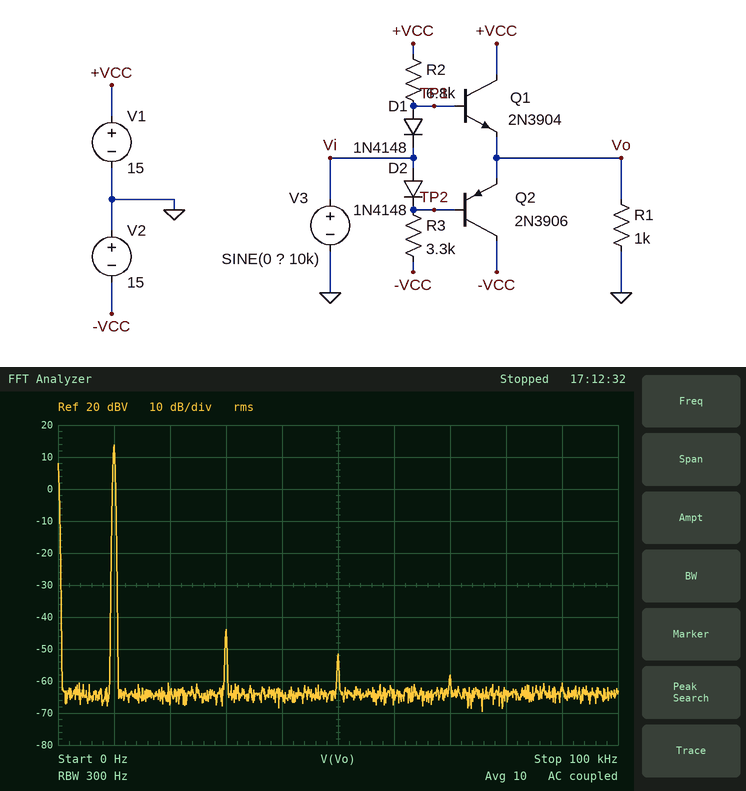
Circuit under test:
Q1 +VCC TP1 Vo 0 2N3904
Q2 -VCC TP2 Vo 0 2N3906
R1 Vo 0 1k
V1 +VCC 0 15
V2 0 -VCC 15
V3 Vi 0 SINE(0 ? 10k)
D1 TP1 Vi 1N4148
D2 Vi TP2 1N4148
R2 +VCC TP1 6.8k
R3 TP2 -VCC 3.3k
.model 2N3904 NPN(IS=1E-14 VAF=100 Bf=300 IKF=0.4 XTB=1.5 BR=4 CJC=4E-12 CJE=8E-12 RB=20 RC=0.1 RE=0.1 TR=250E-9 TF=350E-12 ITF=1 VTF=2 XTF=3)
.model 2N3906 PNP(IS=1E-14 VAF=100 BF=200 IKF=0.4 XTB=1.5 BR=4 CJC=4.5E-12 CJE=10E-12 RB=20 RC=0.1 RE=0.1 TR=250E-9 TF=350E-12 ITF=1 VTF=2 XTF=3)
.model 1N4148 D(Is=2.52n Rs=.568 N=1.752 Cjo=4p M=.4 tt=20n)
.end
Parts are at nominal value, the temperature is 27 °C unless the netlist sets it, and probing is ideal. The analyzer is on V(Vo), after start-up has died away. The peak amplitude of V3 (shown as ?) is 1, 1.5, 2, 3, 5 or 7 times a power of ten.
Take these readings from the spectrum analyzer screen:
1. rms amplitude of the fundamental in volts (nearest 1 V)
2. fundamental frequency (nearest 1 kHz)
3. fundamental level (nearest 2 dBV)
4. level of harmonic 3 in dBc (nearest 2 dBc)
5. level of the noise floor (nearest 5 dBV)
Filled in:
5 V
10 kHz
14 dBV
-58 dBc
-65 dBV
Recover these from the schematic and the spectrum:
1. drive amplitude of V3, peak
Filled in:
7 V
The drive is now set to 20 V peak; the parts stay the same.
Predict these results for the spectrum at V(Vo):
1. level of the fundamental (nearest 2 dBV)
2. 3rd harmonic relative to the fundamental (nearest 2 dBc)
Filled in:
22 dBV
-18 dBc
